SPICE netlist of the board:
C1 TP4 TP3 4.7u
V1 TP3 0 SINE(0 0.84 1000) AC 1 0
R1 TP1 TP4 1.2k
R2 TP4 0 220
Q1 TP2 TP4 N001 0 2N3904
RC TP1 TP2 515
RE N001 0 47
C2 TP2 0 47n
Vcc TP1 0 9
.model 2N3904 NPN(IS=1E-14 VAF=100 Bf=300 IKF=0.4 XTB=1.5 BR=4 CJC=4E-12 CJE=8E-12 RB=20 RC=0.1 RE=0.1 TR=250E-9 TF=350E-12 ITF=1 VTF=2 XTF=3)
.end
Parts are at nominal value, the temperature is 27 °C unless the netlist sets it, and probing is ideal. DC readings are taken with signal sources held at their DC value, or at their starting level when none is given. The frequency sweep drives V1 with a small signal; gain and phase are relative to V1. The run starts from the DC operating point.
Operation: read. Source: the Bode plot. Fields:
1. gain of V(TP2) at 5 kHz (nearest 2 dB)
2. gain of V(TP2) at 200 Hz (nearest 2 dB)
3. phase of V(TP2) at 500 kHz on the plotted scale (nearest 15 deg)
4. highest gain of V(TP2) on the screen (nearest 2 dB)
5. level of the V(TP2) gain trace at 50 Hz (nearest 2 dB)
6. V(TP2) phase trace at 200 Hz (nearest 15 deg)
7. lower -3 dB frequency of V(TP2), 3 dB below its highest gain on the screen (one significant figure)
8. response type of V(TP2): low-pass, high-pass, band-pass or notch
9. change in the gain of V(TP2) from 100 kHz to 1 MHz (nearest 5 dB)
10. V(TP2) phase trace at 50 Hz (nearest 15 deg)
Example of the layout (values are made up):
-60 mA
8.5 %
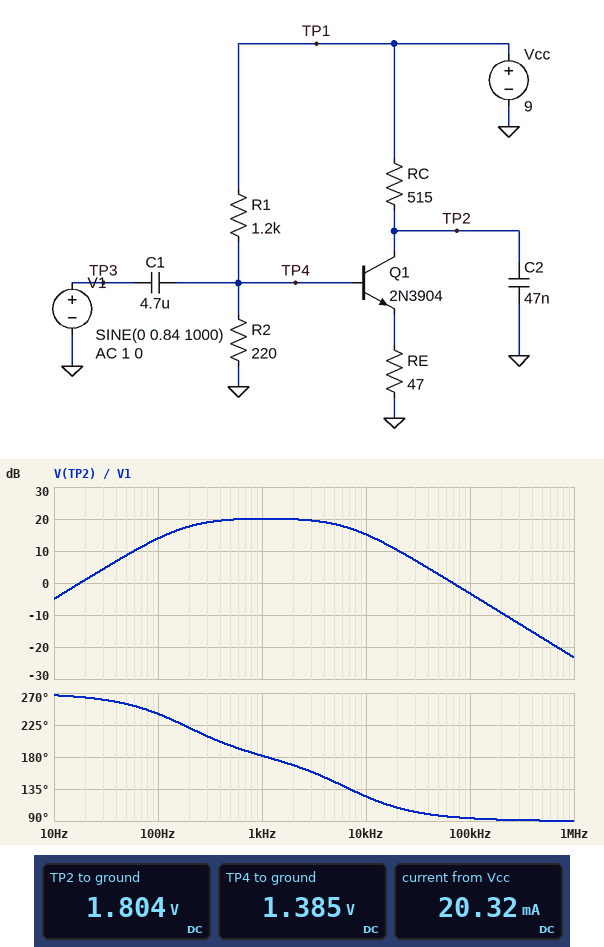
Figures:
18 dB
18 dB
90 deg
20 dB
8 dB
225 deg
200 Hz
band-pass
-20 dB
255 deg
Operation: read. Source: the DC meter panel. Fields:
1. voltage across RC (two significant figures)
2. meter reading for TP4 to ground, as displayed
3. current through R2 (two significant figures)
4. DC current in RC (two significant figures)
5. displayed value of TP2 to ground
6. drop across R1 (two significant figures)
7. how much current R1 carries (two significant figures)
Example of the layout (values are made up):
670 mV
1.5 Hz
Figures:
7.2 V
1.385 V
6.3 mA
14 mA
1.804 V
7.6 V
6.3 mA
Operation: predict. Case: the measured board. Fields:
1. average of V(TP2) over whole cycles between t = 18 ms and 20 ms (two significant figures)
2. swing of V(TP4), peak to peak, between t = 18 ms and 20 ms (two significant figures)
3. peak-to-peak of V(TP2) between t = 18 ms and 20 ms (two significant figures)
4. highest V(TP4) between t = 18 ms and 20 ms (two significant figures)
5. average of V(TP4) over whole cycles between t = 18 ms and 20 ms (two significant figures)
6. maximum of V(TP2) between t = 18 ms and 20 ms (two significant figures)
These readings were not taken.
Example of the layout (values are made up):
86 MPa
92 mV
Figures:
4.8 V
1.6 V
8.2 V
1.9 V
1.1 V
9.0 V
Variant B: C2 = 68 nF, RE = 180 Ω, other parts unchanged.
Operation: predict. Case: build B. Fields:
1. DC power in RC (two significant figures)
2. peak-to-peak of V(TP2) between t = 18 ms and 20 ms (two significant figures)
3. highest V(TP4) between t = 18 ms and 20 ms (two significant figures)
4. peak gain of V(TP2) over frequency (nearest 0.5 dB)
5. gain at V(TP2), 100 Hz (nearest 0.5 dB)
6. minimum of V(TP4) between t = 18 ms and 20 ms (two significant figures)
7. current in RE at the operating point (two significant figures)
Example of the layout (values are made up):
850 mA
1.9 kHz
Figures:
7.8 mW
4.2 V
2.2 V
8.5 dB
2.5 dB
570 mV
3.9 mA
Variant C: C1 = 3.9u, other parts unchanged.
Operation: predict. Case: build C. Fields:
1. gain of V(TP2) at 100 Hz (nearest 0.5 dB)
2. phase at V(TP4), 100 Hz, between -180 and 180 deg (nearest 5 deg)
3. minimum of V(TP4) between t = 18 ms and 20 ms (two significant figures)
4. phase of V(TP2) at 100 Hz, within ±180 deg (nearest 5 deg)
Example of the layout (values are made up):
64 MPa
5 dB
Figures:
12.5 dB
65 deg
330 mV
-115 deg
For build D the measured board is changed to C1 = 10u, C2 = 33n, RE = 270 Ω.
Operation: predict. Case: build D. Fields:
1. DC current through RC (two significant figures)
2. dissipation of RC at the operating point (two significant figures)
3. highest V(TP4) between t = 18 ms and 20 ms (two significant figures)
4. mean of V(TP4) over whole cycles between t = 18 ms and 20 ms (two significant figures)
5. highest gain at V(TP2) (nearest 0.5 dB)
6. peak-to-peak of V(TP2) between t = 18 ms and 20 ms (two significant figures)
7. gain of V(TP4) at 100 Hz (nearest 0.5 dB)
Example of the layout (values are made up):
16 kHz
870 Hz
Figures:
2.6 mA
3.6 mW
2.2 V
1.4 V
5.0 dB
2.9 V
-2.5 dB
